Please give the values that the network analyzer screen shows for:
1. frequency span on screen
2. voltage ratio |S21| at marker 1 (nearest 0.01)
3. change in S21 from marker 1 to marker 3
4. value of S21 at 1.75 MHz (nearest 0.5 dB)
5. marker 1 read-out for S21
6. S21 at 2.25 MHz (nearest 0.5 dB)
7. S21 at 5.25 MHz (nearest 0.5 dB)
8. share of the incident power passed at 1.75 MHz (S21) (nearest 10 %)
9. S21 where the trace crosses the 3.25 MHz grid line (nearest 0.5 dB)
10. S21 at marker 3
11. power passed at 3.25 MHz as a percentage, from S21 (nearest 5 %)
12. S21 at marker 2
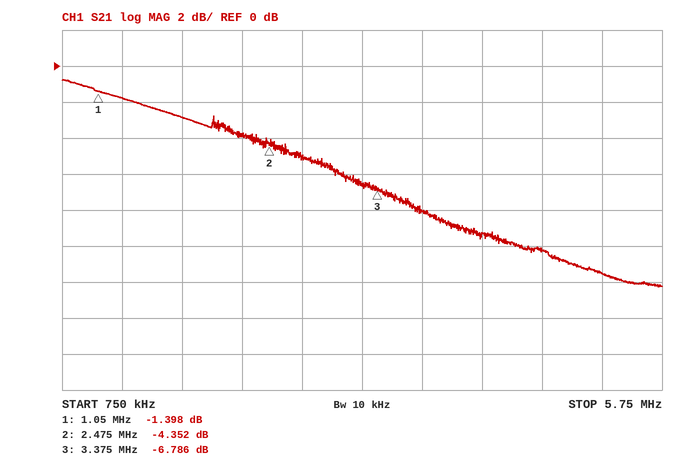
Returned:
5 MHz
0.85
-5.388 dB
-3.0 dB
-1.398 dB
-4.0 dB
-11.5 dB
50 %
-6.5 dB
-6.786 dB
20 %
-4.352 dB
